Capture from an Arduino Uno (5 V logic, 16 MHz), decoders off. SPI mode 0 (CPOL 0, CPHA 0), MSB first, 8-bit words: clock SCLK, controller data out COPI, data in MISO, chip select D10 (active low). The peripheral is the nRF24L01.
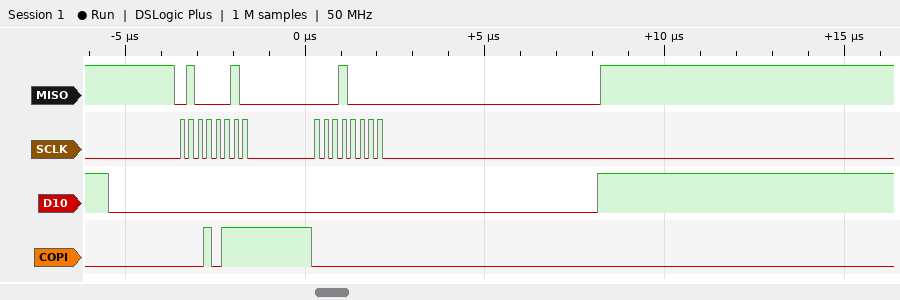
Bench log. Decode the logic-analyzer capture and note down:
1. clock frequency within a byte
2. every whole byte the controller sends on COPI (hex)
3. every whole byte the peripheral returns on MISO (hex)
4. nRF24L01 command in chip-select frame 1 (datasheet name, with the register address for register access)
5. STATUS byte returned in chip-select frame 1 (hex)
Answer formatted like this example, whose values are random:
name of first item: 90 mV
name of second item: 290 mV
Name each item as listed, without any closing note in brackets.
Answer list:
clock frequency within a byte: 4 MHz
every whole byte the controller sends on COPI: 0x17 0x00
every whole byte the peripheral returns on MISO: 0x42 0x10
nRF24L01 command in chip-select frame 1: R_REGISTER 0x17
STATUS byte returned in chip-select frame 1: 0x42
